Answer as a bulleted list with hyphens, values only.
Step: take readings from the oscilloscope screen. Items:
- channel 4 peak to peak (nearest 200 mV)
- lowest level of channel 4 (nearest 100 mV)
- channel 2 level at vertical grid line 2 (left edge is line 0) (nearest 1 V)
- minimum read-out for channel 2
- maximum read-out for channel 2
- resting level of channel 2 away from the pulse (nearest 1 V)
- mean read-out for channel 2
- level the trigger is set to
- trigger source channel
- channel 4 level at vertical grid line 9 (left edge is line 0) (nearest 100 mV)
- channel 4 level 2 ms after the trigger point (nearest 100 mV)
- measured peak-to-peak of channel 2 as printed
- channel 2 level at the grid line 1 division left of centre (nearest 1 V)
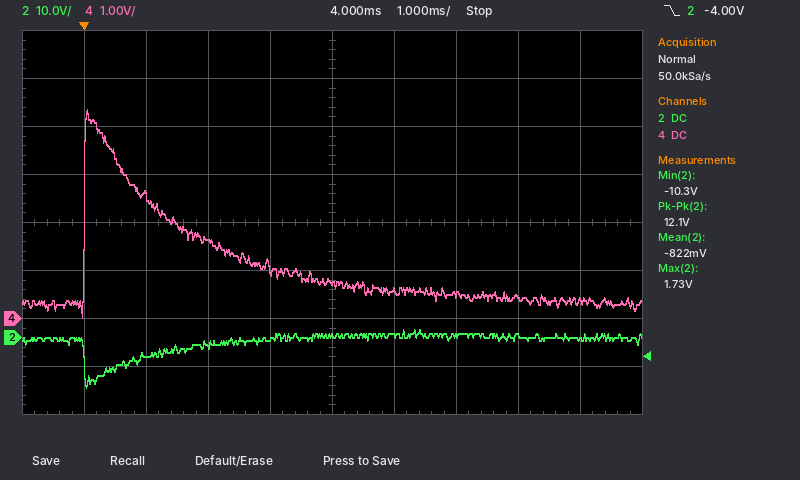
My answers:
- 4.4 V
- 0.0 V
- -4 V
- -10.3 V
- 1.73 V
- 0 V
- -822 mV
- -4.00 V
- channel 2
- 400 mV
- 1.6 V
- 12.1 V
- 0 V
